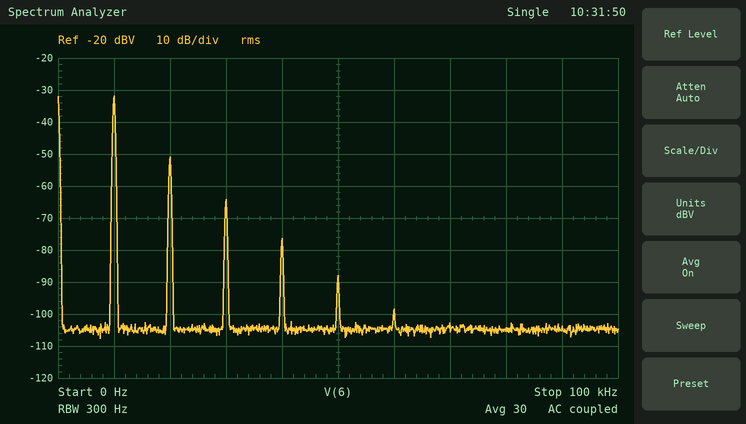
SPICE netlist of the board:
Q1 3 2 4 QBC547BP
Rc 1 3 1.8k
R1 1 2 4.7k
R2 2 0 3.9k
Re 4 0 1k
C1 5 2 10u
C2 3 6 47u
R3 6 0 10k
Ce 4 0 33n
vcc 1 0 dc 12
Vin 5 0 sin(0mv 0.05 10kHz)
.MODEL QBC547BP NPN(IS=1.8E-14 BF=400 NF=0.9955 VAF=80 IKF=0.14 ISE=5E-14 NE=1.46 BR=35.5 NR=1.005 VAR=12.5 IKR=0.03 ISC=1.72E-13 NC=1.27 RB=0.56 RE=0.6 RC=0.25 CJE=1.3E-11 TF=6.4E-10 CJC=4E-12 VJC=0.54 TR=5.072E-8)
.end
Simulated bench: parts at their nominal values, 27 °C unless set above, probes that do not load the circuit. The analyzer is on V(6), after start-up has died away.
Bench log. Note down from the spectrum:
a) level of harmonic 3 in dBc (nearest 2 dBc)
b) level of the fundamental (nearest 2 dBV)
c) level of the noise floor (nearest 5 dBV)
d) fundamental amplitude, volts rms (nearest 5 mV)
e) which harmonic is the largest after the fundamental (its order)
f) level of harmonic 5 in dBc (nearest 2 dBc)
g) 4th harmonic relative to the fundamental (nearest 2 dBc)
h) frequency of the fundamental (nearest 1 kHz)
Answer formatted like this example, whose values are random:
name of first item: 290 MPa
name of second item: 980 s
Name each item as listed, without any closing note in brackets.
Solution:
level of harmonic 3 in dBc: -32 dBc
level of the fundamental: -32 dBV
level of the noise floor: -105 dBV
fundamental amplitude, volts rms: 25 mV
which harmonic is the largest after the fundamental: 2
level of harmonic 5 in dBc: -56 dBc
4th harmonic relative to the fundamental: -44 dBc
frequency of the fundamental: 10 kHz
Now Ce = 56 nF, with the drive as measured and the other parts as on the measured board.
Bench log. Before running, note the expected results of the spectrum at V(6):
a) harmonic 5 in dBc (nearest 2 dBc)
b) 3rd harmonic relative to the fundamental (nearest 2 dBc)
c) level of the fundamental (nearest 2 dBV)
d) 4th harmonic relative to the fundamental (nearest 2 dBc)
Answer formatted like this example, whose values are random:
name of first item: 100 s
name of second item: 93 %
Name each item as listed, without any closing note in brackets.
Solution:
harmonic 5 in dBc: -34 dBc
3rd harmonic relative to the fundamental: -20 dBc
level of the fundamental: -30 dBV
4th harmonic relative to the fundamental: -28 dBc
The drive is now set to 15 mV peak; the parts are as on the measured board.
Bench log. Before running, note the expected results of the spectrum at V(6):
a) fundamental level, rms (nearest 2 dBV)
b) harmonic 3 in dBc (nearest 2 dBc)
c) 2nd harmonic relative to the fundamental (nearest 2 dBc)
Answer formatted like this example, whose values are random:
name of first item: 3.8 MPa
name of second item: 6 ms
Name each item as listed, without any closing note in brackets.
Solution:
fundamental level, rms: -42 dBV
harmonic 3 in dBc: -56 dBc
2nd harmonic relative to the fundamental: -32 dBc
